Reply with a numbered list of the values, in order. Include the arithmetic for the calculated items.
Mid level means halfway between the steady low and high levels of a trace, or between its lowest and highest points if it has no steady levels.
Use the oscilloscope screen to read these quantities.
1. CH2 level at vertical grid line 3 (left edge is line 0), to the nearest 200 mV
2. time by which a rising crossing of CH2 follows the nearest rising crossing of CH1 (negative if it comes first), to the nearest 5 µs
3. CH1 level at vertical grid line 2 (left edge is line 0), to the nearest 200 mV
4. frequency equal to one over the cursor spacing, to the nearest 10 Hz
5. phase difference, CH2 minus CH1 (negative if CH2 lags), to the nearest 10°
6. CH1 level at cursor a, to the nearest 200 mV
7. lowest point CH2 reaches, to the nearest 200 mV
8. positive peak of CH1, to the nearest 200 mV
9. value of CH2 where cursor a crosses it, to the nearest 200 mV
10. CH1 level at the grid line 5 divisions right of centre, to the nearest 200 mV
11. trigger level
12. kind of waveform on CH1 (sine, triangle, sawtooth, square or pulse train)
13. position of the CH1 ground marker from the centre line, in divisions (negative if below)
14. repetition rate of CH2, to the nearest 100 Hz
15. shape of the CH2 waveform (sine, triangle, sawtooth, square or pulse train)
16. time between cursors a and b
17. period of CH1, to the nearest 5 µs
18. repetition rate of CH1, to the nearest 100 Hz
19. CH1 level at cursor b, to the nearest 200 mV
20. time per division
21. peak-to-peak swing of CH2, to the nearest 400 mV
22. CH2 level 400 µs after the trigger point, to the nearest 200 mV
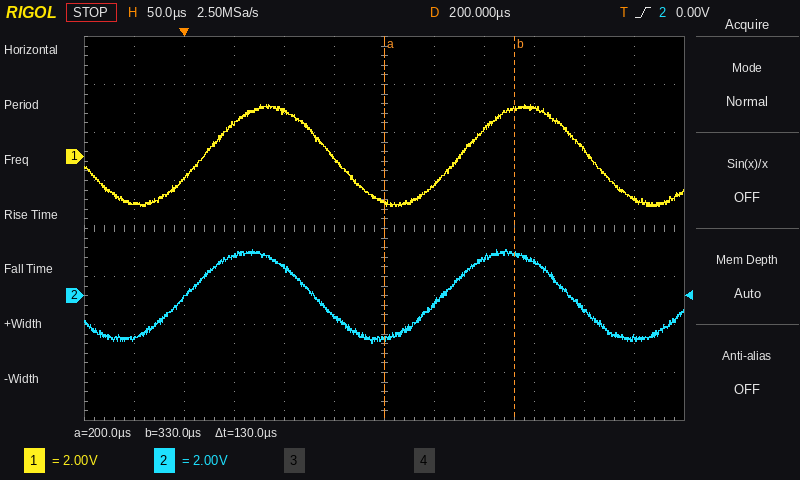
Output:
1. 1.6 V
2. -20 µs
3. -800 mV
4. 1 / 130 µs ≈ 7.69 kHz
5. −360° × (-20 µs) / 255 µs ≈ +28.2°, so +30° to the nearest 10°
6. -2.0 V
7. -2.0 V
8. 2.2 V
9. -1.8 V
10. -1.8 V
11. 0.00 V
12. sine
13. +1.5 div
14. 3.9 kHz
15. sine
16. 130 µs
17. 255 µs
18. 1 / 255 µs ≈ 3.9 kHz
19. 2.0 V
20. 50 µs
21. 4.0 V
22. -600 mV
